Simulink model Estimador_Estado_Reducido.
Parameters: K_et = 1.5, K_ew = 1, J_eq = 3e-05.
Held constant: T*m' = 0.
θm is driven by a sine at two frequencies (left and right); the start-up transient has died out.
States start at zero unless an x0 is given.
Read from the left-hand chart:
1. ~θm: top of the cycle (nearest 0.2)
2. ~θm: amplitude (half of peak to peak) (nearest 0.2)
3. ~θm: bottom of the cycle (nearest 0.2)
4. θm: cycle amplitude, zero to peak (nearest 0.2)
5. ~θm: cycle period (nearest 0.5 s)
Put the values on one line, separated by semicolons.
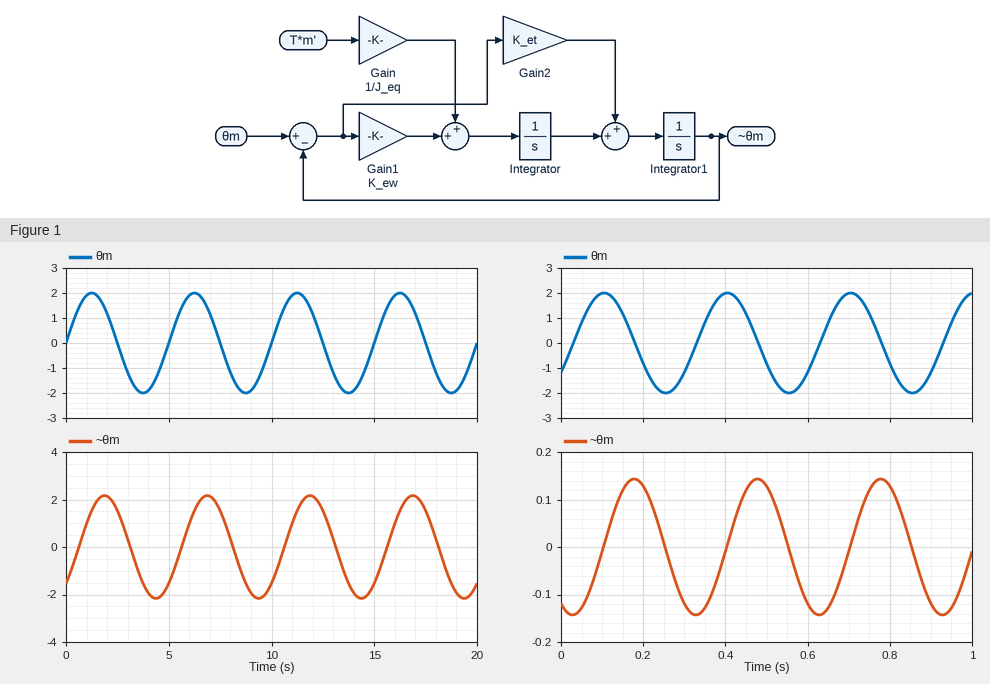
2.2; 2.2; -2.2; 2.0; 5.0 s
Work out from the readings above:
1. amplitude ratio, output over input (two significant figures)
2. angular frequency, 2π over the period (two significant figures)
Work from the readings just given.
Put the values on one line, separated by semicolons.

1.1; 1.3 rad/s
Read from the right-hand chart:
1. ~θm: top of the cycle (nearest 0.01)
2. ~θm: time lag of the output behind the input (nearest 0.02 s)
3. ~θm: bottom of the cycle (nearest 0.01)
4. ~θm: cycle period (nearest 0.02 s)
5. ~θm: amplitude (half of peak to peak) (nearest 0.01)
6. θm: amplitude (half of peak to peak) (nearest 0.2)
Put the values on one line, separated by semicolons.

0.14; 0.08 s; -0.14; 0.30 s; 0.14; 2.0
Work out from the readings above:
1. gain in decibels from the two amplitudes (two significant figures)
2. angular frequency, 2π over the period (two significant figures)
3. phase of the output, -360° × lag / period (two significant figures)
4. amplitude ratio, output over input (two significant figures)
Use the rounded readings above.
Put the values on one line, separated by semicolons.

-23 dB; 21 rad/s; -96°; 0.070
